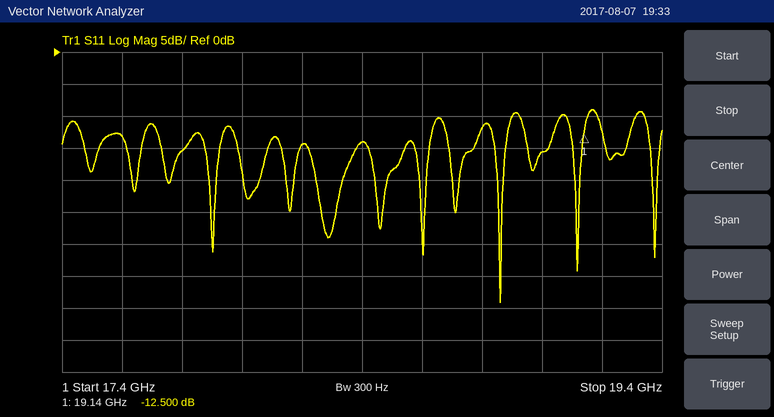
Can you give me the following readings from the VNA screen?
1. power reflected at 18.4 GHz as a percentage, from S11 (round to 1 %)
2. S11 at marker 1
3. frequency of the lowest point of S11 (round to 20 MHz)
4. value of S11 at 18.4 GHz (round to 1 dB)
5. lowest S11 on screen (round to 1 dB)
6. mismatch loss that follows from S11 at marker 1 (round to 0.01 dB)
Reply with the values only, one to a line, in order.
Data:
4 %
-12.500 dB
18.86 GHz
-14 dB
-39 dB
0.25 dB
